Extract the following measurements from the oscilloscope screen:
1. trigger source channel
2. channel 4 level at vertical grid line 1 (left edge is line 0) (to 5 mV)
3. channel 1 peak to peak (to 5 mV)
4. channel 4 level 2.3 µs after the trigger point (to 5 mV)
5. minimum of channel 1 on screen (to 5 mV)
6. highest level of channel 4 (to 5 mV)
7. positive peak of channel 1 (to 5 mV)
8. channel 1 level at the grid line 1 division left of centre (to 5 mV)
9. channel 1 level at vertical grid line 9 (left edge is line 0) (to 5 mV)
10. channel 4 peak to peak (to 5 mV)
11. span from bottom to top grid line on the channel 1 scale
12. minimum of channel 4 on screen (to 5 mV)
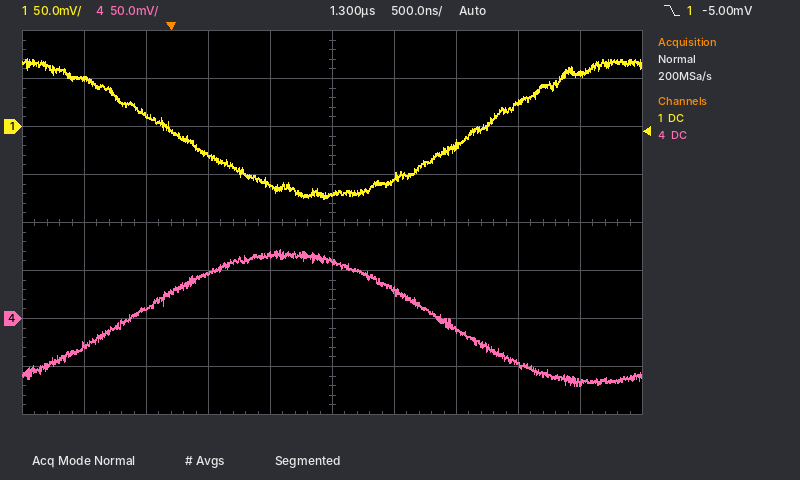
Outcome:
channel 1
-30 mV
145 mV
-10 mV
-75 mV
70 mV
70 mV
-60 mV
55 mV
140 mV
400 mV
-70 mV
